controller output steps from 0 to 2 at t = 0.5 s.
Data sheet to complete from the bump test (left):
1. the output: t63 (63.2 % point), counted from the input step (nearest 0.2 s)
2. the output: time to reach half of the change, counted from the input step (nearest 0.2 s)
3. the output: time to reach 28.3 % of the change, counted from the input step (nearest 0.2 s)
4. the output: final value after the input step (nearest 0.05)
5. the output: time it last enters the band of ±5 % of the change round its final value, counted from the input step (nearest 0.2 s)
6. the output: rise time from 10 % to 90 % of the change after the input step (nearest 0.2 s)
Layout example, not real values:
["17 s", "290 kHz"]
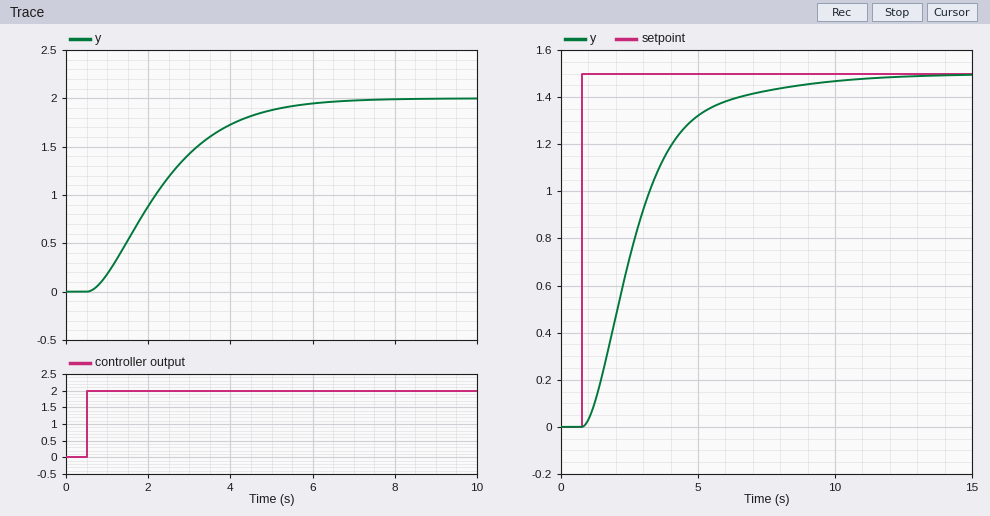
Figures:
["2.2 s", "1.6 s", "1.0 s", "2.00", "4.8 s", "3.4 s"]
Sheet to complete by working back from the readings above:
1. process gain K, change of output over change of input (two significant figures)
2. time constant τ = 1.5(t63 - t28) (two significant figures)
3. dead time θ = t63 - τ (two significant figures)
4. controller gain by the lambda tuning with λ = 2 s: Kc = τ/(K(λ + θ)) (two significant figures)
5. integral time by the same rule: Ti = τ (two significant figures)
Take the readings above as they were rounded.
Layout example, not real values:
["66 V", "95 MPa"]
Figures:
["1.0", "1.8 s", "0.40 s", "0.75", "1.8 s"]
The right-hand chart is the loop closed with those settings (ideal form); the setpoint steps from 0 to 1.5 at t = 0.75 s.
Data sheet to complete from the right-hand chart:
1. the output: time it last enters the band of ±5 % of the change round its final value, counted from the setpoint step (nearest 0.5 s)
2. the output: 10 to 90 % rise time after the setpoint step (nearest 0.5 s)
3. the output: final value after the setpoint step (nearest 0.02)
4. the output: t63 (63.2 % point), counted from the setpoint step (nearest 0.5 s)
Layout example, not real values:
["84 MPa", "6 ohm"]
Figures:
["6.5 s", "4.0 s", "1.50", "2.5 s"]
